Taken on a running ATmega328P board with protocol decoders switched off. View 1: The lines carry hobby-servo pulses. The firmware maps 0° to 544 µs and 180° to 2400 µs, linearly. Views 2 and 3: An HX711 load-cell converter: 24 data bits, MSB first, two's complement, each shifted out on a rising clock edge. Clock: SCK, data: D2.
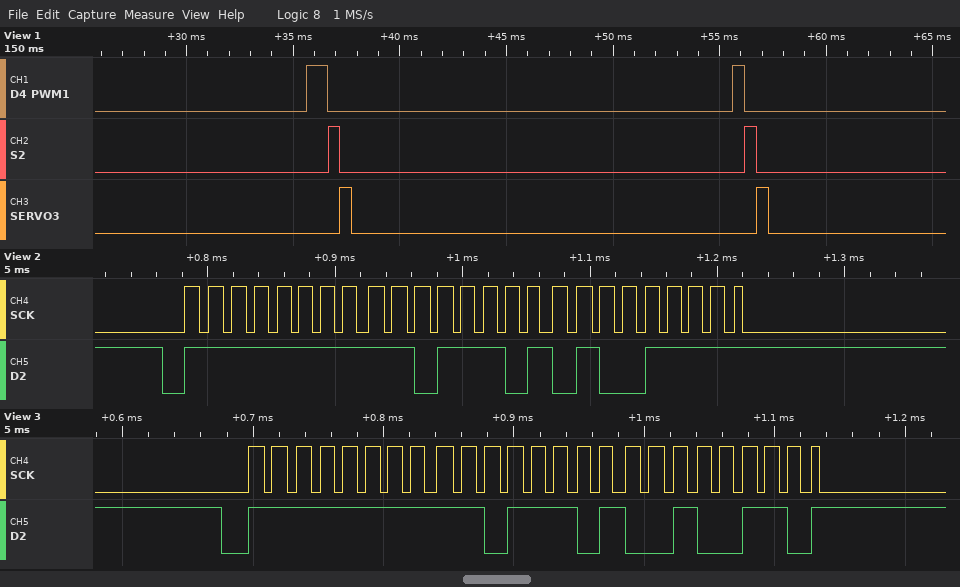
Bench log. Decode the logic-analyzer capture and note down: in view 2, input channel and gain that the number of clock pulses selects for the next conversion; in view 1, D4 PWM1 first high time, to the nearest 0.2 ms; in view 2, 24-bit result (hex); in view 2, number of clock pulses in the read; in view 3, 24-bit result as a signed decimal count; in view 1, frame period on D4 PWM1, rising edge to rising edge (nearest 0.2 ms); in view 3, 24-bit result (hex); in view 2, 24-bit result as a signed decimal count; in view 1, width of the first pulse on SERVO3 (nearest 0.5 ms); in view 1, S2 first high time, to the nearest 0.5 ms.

channel A, gain 128
1.0 ms
0xFFDD4F
25
-8922
20.0 ms
0xFFDD26
-8881
0.5 ms
0.5 ms
